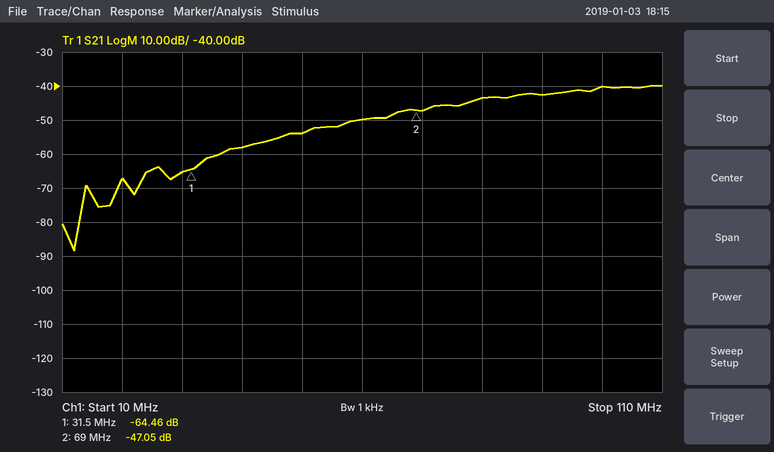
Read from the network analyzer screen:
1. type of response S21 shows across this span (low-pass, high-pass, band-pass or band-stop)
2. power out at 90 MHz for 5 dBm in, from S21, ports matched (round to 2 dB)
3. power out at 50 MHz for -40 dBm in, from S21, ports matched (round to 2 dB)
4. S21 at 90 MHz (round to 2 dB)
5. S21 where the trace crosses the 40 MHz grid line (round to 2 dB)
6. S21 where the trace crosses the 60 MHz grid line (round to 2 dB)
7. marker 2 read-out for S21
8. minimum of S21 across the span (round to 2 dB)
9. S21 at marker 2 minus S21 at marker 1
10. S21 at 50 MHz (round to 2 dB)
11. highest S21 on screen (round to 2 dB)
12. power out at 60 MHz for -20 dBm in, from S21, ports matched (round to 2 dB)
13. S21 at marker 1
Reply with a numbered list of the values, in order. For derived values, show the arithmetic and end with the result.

1. high-pass
2. 5 dBm + (-42 dB) = -38 dBm
3. -40 dBm + (-54 dB) = -94 dBm
4. -42 dB
5. -58 dB
6. -50 dB
7. -47.05 dB
8. -88 dB
9. -47.05 − (-64.46) = 17.41 dB
10. -54 dB
11. -40 dB
12. -20 dBm + (-50 dB) = -70 dBm
13. -64.46 dB
